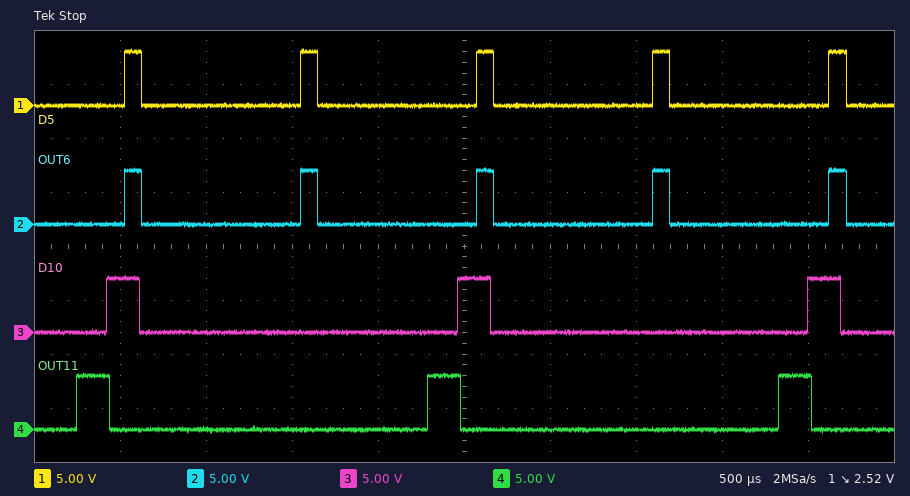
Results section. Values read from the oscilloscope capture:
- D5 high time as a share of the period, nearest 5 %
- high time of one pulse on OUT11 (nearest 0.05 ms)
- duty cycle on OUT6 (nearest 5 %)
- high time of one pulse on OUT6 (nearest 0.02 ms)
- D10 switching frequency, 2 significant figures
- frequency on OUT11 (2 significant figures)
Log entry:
10 %
0.20 ms
10 %
0.10 ms
490 Hz
490 Hz
